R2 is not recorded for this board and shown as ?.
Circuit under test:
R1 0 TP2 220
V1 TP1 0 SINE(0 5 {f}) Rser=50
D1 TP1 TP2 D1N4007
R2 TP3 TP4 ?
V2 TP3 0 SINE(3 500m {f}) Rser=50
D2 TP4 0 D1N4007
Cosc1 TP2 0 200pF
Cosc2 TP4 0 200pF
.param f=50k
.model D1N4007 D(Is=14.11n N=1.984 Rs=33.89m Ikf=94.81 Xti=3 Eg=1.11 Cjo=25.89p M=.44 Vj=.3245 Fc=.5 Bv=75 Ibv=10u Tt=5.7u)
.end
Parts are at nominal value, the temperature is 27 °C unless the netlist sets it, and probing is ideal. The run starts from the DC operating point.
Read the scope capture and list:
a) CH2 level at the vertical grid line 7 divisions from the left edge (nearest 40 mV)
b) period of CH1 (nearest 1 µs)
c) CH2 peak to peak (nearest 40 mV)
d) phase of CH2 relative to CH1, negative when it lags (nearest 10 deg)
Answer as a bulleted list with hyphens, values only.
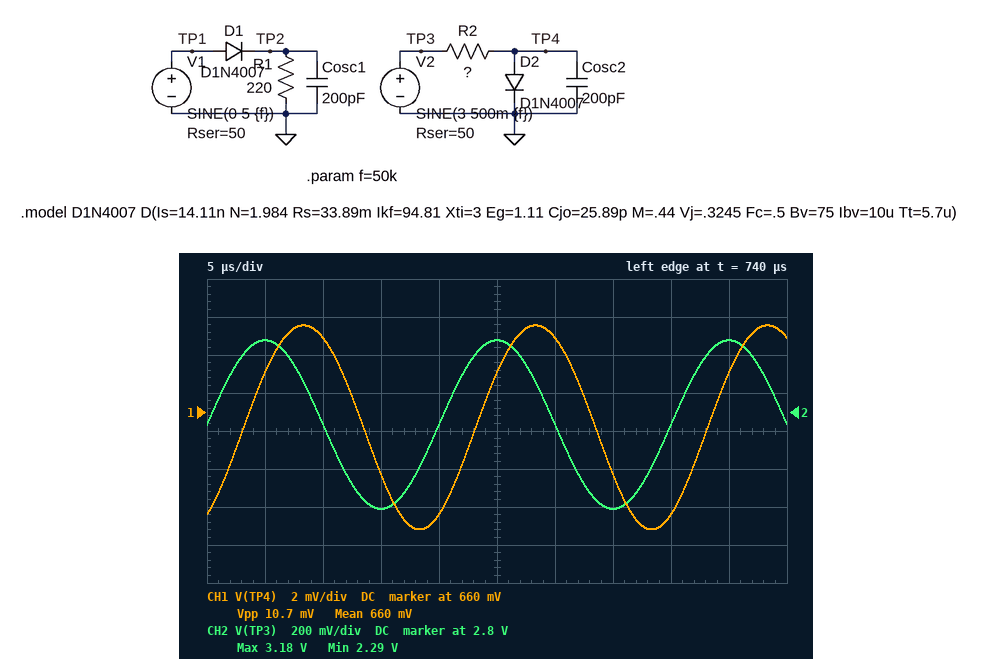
- 2.28 V
- 20 µs
- 880 mV
- 60 deg
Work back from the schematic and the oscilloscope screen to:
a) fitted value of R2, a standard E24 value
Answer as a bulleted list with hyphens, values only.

- 390 Ω
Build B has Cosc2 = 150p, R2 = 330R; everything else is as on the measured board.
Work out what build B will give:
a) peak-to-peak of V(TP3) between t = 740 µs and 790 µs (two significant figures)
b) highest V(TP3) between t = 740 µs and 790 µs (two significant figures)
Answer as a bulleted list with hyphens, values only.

- 870 mV
- 3.1 V
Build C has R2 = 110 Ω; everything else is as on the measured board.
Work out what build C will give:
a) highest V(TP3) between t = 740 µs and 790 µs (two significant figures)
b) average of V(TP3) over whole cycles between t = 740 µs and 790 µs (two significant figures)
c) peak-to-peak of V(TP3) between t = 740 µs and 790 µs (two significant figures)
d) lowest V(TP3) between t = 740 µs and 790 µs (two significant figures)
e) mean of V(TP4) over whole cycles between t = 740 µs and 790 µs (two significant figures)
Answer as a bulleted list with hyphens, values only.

- 2.6 V
- 2.3 V
- 690 mV
- 1.9 V
- 710 mV
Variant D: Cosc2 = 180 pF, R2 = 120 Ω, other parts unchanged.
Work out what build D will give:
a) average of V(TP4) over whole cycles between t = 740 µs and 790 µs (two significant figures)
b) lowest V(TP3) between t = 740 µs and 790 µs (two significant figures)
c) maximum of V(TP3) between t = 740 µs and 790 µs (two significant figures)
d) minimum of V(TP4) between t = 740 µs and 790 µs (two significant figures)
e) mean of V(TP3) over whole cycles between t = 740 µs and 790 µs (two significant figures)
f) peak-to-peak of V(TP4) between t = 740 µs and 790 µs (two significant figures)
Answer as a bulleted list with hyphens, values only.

- 710 mV
- 2.0 V
- 2.7 V
- 700 mV
- 2.3 V
- 11 mV
